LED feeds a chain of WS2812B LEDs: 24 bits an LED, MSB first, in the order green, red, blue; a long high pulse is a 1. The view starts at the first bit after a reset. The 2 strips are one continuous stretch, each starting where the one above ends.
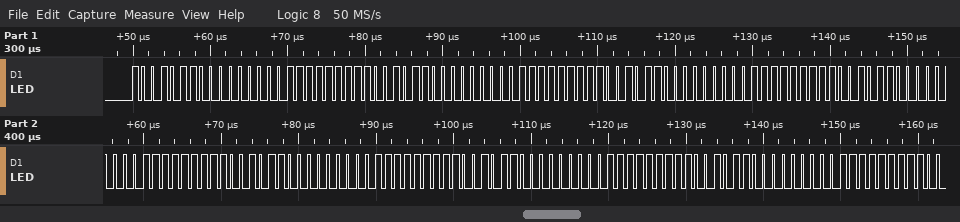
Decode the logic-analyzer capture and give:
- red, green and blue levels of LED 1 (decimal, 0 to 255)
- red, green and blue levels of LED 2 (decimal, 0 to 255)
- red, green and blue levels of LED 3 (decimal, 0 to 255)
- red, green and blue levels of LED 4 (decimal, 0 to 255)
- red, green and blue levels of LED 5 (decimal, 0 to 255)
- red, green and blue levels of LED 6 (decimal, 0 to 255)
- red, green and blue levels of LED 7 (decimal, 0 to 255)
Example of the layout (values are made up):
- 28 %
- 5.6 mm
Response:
- 0, 150, 255
- 0, 150, 255
- 0, 150, 255
- 0, 150, 255
- 0, 150, 255
- 0, 150, 255
- 0, 150, 255
